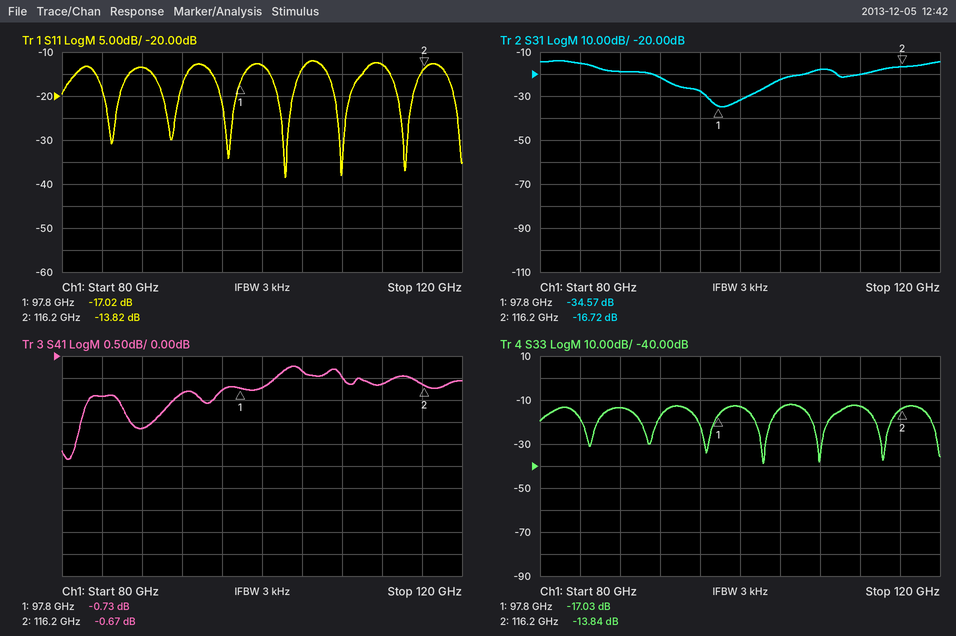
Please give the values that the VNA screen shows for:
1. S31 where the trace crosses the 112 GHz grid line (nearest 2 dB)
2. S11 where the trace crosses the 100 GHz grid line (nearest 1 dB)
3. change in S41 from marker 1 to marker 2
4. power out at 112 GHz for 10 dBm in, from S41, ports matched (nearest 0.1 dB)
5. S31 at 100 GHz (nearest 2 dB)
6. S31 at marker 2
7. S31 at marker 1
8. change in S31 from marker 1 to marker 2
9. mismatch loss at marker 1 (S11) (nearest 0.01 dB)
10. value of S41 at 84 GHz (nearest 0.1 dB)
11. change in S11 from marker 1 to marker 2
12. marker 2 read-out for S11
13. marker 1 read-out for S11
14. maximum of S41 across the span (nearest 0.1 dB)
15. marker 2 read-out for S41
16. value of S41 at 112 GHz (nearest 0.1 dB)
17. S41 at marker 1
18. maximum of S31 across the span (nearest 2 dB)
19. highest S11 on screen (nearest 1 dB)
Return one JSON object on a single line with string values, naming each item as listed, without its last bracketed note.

{"S31 where the trace crosses the 112 GHz grid line": "-20 dB", "S11 where the trace crosses the 100 GHz grid line": "-13 dB", "change in S41 from marker 1 to marker 2": "0.06 dB", "power out at 112 GHz for 10 dBm in, from S41, ports matched": "9.4 dBm", "S31 at 100 GHz": "-32 dB", "S31 at marker 2": "-16.72 dB", "S31 at marker 1": "-34.57 dB", "change in S31 from marker 1 to marker 2": "17.85 dB", "mismatch loss at marker 1 (S11)": "0.09 dB", "value of S41 at 84 GHz": "-0.9 dB", "change in S11 from marker 1 to marker 2": "3.20 dB", "marker 2 read-out for S11": "-13.82 dB", "marker 1 read-out for S11": "-17.02 dB", "maximum of S41 across the span": "-0.2 dB", "marker 2 read-out for S41": "-0.67 dB", "value of S41 at 112 GHz": "-0.6 dB", "S41 at marker 1": "-0.73 dB", "maximum of S31 across the span": "-14 dB", "highest S11 on screen": "-12 dB"}
